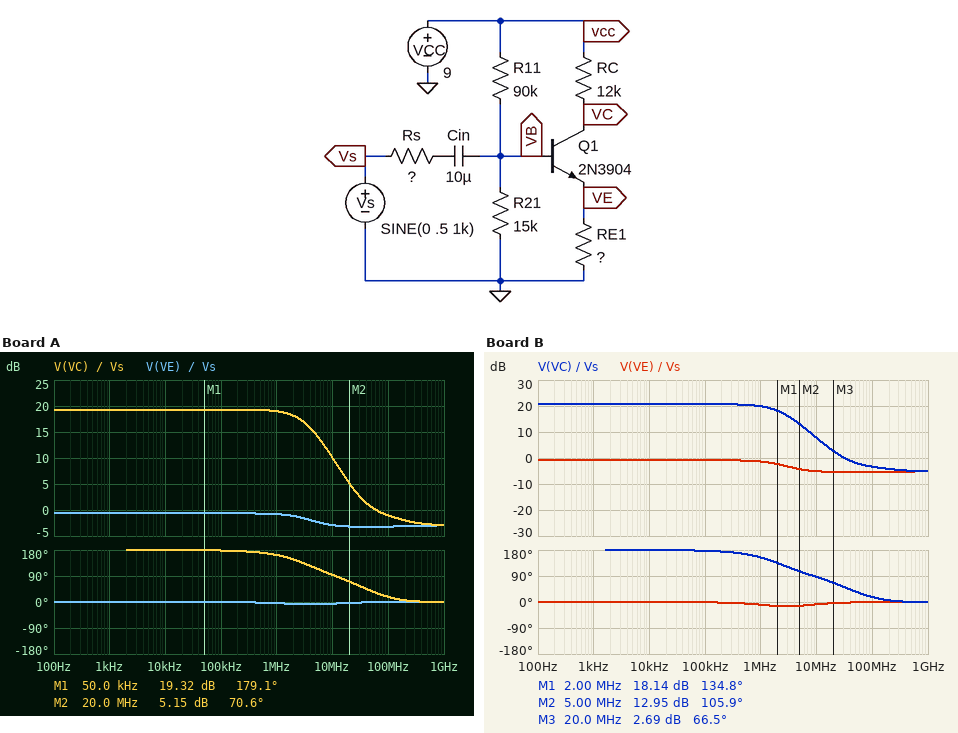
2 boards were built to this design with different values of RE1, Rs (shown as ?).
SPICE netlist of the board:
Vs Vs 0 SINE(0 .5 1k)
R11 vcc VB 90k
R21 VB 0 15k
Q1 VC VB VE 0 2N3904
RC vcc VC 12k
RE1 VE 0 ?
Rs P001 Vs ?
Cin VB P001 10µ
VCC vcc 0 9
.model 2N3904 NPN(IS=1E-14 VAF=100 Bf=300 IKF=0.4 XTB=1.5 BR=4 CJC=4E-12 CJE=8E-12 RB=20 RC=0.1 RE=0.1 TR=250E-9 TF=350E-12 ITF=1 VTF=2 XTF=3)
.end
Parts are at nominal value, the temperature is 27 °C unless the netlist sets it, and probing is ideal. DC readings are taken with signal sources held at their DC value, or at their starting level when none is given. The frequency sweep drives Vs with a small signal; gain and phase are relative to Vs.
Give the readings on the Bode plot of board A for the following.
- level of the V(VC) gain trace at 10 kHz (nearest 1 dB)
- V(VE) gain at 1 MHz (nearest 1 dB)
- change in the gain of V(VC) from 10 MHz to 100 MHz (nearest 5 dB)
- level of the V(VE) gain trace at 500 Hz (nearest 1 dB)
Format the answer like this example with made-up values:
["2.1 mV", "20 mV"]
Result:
["19 dB", "-1 dB", "-10 dB", "-1 dB"]
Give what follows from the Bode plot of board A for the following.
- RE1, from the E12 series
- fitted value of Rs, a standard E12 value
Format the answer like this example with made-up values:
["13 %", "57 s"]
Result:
["1.2 kΩ", "390 Ω"]
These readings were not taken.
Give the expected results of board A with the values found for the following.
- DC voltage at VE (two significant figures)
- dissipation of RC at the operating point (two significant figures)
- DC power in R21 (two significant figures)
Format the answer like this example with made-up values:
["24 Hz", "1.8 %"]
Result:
["630 mV", "3.2 mW", "110 µW"]
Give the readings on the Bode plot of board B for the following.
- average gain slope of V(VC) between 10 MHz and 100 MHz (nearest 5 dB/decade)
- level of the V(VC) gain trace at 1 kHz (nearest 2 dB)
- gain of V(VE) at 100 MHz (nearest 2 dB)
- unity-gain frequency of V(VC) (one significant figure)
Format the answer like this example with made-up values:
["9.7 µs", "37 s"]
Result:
["-10 dB/decade", "20 dB", "-6 dB", "30 MHz"]
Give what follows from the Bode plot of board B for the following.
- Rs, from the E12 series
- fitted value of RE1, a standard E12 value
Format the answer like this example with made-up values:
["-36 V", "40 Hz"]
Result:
["680 Ω", "1 kΩ"]
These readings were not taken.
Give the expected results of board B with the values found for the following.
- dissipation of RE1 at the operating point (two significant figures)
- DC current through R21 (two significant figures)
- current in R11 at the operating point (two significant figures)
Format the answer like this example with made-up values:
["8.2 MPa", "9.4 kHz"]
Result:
["380 µW", "84 µA", "86 µA"]
